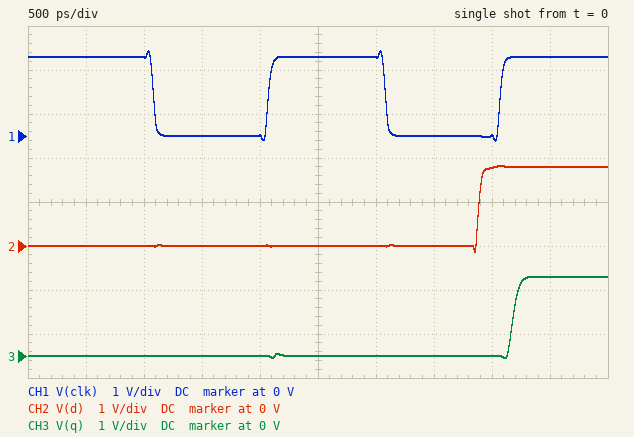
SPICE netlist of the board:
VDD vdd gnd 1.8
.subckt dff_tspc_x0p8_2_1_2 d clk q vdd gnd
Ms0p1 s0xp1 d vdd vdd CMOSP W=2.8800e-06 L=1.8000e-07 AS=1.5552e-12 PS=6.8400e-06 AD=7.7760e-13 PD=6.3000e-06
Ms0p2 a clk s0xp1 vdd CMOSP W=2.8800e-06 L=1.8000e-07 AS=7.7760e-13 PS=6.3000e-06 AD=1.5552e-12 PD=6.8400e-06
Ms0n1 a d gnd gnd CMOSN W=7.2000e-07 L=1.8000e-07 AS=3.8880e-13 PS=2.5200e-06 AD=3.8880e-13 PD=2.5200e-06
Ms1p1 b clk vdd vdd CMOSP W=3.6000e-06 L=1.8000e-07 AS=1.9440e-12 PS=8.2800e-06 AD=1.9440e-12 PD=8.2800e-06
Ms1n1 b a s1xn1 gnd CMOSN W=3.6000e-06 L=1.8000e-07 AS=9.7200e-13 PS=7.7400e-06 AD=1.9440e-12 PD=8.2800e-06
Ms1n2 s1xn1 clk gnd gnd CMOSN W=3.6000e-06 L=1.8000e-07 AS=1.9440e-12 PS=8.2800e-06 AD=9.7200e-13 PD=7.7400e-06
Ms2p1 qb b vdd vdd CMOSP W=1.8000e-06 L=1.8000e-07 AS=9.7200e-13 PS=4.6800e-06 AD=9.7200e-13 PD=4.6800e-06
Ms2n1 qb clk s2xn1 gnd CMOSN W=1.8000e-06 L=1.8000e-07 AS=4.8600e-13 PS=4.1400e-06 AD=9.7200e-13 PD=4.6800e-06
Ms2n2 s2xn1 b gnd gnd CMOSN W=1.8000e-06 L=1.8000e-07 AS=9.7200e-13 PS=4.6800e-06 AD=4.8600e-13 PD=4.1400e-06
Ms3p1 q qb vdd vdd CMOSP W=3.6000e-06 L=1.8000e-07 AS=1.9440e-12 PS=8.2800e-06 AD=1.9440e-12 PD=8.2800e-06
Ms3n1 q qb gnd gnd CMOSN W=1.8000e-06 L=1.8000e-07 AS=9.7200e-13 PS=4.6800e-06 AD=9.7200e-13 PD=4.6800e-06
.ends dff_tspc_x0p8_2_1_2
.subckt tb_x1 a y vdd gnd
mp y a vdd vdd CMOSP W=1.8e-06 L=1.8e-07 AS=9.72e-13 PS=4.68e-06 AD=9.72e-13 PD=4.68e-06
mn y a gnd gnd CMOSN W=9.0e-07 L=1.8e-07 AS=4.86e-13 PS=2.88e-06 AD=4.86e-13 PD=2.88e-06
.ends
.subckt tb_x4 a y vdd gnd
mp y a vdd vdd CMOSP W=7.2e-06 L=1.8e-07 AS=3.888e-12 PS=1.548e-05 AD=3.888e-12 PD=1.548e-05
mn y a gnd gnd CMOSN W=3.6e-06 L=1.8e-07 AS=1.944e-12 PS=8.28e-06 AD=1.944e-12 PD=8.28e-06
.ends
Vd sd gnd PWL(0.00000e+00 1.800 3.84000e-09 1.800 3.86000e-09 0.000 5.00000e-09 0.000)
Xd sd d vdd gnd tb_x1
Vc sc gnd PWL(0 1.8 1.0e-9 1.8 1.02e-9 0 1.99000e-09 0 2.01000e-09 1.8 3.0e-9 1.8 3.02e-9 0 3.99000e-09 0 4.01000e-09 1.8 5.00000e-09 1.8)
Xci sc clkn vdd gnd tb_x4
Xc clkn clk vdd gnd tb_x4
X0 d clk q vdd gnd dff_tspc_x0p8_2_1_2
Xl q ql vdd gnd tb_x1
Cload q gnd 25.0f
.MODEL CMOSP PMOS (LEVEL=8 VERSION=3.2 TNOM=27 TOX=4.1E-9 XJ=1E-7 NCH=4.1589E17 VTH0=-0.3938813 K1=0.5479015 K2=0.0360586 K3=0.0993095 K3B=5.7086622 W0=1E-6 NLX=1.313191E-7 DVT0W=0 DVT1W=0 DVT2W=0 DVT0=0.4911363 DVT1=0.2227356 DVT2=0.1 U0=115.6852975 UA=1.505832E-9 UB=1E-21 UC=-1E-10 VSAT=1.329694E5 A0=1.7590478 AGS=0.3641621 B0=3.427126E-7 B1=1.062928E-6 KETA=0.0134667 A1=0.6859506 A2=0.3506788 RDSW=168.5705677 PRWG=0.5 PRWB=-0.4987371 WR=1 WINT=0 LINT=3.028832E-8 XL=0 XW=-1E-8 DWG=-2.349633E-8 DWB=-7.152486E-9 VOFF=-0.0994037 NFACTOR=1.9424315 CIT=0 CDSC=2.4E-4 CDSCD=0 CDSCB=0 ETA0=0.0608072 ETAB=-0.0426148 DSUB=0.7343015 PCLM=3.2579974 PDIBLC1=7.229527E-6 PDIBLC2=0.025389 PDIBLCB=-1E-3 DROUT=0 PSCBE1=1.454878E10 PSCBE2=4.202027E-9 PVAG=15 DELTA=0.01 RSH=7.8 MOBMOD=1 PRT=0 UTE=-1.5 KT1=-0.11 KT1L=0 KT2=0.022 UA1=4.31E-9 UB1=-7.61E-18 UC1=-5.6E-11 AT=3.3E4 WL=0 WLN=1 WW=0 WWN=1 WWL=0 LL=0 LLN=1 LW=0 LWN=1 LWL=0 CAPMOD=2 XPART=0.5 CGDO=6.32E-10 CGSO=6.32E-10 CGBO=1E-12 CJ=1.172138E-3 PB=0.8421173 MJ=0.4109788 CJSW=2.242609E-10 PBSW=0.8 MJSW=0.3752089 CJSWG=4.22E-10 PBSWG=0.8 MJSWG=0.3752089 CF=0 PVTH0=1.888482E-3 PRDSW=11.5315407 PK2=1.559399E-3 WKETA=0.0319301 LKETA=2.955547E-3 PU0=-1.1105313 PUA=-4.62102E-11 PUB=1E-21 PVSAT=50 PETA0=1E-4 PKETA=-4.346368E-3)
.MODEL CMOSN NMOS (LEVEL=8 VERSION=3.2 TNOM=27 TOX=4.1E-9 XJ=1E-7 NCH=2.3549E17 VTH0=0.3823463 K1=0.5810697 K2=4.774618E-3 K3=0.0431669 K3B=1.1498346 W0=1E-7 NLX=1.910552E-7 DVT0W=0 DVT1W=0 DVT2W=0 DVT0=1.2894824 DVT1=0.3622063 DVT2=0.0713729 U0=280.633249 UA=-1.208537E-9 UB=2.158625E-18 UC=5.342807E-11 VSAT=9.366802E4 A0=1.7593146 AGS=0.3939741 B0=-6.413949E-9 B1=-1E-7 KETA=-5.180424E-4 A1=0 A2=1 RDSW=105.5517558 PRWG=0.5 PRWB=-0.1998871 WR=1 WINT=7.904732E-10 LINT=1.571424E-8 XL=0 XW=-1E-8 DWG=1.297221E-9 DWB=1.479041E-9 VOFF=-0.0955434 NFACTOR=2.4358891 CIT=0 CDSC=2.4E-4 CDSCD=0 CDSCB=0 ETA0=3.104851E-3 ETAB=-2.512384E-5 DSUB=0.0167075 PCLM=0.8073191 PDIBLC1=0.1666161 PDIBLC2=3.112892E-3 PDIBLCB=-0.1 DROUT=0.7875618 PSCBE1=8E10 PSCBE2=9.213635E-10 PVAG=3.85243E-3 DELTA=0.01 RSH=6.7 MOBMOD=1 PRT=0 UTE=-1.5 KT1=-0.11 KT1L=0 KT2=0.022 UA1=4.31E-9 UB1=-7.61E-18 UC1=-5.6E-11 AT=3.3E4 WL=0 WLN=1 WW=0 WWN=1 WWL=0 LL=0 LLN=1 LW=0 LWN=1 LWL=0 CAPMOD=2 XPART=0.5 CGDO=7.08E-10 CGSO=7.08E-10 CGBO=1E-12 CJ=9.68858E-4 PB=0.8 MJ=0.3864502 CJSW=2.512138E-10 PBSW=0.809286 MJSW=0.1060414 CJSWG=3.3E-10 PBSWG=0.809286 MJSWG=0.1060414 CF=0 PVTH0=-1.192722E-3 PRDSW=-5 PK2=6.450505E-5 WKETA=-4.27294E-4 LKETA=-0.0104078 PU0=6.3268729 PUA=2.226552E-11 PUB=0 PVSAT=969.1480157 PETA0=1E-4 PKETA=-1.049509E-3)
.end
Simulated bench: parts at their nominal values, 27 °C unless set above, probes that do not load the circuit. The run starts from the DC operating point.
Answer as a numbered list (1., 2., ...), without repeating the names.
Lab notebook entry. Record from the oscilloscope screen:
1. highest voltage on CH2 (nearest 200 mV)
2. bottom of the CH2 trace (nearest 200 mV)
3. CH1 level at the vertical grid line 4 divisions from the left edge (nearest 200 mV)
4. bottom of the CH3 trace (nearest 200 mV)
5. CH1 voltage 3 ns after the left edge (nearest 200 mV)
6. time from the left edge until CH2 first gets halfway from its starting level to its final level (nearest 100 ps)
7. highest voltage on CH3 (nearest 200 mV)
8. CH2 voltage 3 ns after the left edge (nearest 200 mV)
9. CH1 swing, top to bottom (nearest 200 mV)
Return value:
1. 1.8 V
2. -200 mV
3. 0 V
4. 0 V
5. 1.8 V
6. 3.9 ns
7. 1.8 V
8. 0 V
9. 2.0 V
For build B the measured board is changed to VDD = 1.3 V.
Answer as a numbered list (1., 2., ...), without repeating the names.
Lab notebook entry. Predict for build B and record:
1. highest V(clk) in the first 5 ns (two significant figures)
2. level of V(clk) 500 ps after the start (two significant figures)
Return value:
1. 1.4 V
2. 1.3 V
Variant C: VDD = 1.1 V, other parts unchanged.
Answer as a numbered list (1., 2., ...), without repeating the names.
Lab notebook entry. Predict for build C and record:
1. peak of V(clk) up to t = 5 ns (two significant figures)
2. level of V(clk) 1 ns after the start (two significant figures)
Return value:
1. 1.2 V
2. 1.1 V
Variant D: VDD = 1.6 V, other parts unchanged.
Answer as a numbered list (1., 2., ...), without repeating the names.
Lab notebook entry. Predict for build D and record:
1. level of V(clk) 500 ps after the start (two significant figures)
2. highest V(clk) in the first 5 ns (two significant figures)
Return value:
1. 1.6 V
2. 1.7 V
